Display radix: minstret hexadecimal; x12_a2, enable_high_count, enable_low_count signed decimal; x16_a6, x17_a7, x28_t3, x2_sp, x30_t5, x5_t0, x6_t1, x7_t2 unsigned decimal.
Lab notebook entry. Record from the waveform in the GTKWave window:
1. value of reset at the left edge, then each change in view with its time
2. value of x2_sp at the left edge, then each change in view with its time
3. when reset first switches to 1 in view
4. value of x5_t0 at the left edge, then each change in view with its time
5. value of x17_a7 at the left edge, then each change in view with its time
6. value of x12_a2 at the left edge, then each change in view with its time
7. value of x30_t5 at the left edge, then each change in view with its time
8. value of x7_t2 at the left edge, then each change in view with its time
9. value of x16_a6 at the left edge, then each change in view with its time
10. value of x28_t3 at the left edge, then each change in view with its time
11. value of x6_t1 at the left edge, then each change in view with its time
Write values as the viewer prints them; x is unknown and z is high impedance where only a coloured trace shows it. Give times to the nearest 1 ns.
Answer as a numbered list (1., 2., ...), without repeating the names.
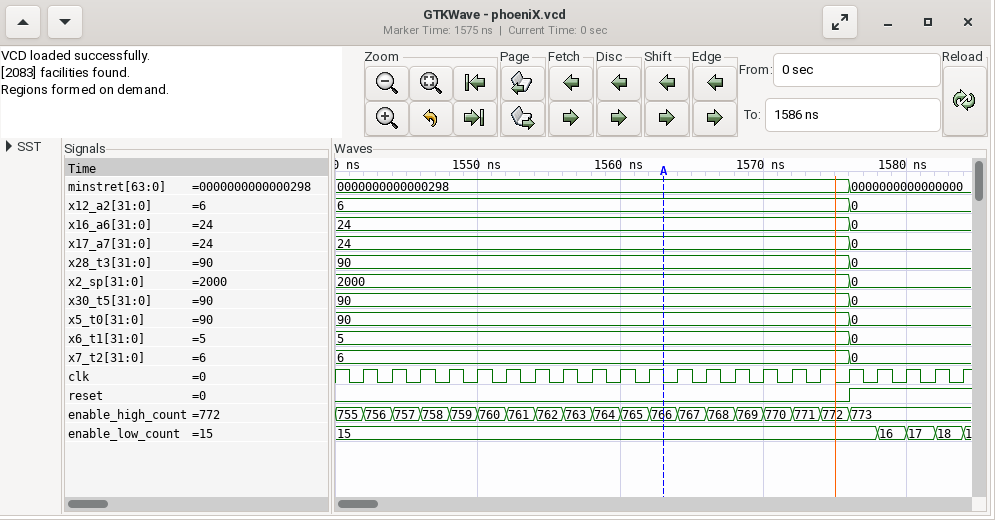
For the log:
1. 0, 1 at 1576 ns
2. 2000, 0 at 1576 ns
3. 1576 ns
4. 90, 0 at 1576 ns
5. 24, 0 at 1576 ns
6. 6, 0 at 1576 ns
7. 90, 0 at 1576 ns
8. 6, 0 at 1576 ns
9. 24, 0 at 1576 ns
10. 90, 0 at 1576 ns
11. 5, 0 at 1576 ns
